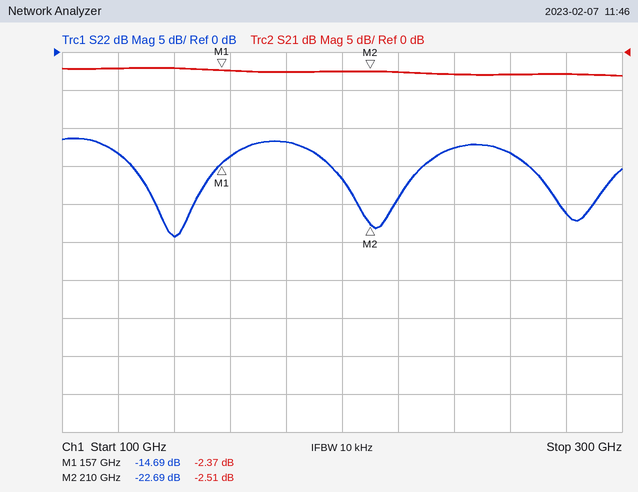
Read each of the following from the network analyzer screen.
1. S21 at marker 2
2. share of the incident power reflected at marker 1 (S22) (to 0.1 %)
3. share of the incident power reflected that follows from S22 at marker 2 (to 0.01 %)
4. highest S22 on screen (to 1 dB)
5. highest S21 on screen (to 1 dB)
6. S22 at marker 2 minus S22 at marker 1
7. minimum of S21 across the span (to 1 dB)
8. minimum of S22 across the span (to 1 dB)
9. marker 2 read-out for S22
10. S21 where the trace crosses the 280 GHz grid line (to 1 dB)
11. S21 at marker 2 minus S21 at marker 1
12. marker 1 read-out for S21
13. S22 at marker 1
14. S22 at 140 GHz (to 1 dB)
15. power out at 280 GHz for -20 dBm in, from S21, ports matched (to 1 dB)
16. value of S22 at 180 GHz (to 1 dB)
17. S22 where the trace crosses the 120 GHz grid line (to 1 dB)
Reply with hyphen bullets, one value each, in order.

- -2.51 dB
- 3.4 %
- 0.54 %
- -11 dB
- -2 dB
- -8.00 dB
- -3 dB
- -24 dB
- -22.69 dB
- -3 dB
- -0.14 dB
- -2.37 dB
- -14.69 dB
- -24 dB
- -23 dBm
- -12 dB
- -13 dB
